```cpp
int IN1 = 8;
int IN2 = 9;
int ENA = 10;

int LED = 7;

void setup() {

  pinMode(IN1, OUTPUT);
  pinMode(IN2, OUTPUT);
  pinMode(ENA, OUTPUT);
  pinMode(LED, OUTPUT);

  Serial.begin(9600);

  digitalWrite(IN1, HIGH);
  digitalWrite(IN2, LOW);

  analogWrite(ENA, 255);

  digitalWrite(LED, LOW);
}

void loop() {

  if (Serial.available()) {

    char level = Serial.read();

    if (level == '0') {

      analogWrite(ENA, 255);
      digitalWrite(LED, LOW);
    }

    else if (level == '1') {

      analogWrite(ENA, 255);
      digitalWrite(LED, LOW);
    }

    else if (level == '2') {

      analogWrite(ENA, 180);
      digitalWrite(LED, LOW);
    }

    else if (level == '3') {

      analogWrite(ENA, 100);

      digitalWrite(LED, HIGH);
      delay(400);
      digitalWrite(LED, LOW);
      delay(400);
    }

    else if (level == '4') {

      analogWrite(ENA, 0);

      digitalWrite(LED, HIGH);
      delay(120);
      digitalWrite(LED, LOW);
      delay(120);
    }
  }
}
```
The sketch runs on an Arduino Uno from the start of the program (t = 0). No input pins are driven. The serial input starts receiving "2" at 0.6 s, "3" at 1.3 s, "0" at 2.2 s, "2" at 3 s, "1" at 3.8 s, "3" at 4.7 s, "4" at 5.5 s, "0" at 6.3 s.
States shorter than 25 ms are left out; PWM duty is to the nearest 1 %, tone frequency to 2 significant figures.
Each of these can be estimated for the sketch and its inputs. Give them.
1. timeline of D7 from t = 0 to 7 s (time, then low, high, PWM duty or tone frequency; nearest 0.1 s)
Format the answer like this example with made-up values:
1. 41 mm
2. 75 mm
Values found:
1. 0 s low; 1.3 s high; 1.7 s low; 4.7 s high; 5.1 s low; 5.5 s high; 5.6 s low
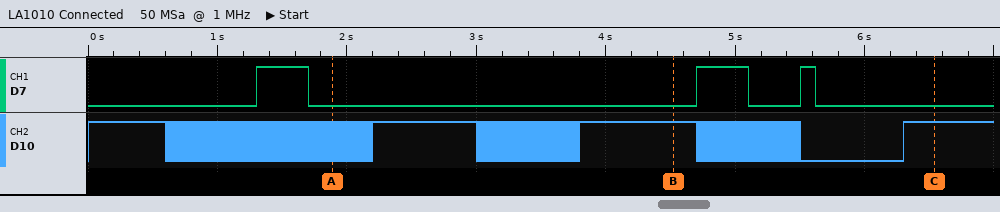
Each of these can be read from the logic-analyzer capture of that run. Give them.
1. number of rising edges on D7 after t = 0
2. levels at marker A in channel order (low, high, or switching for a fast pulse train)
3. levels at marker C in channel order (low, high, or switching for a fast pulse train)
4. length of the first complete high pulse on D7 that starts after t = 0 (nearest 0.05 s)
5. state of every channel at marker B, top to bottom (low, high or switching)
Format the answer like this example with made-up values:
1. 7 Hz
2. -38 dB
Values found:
1. 3
2. D7 low, D10 switching
3. D7 low, D10 high
4. 0.40 s
5. D7 low, D10 high
